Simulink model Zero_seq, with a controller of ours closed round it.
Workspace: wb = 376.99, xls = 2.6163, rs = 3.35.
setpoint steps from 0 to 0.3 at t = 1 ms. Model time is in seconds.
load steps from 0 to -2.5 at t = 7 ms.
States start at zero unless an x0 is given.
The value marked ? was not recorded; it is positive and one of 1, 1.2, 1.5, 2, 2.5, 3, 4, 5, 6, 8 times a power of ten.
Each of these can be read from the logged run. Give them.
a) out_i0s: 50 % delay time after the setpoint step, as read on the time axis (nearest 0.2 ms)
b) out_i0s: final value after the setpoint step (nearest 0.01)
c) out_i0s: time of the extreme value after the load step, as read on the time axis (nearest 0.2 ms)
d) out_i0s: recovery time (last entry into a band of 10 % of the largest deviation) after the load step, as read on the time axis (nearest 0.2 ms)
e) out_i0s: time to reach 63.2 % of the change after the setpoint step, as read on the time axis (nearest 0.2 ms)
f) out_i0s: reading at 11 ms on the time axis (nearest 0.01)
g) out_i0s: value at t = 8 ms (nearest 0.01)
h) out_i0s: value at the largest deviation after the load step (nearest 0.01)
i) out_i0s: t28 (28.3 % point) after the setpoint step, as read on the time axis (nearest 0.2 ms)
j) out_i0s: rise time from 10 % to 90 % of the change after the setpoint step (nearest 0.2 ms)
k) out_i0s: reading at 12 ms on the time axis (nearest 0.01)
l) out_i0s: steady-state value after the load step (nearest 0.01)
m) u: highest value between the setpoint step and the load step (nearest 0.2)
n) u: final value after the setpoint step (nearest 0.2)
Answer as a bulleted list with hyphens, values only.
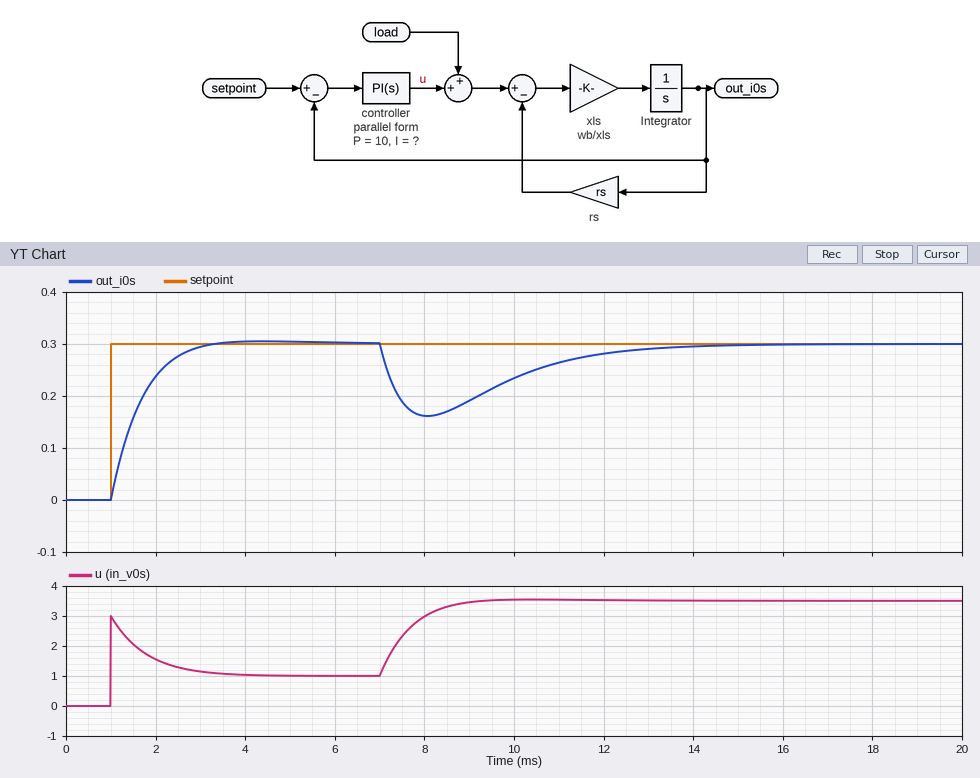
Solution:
- 1.4 ms
- 0.30
- 8.0 ms
- 12.4 ms
- 1.6 ms
- 0.26
- 0.16
- 0.16
- 1.2 ms
- 1.4 ms
- 0.28
- 0.30
- 3.0
- 1.0
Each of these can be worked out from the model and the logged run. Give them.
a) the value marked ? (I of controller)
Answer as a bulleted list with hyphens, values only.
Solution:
- 6000
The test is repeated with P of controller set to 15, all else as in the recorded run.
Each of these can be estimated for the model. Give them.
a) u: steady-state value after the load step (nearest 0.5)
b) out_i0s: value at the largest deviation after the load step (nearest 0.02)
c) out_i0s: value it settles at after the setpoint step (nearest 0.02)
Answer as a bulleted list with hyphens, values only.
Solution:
- 3.5
- 0.18
- 0.30
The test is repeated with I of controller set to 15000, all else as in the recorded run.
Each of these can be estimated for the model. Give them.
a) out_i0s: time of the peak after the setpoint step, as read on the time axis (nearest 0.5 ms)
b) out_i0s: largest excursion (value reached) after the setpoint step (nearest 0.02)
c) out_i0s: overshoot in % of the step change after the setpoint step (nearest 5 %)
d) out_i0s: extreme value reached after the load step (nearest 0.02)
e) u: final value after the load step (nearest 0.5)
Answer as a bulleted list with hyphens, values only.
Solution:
- 3.0 ms
- 0.34
- 15 %
- 0.18
- 3.5
